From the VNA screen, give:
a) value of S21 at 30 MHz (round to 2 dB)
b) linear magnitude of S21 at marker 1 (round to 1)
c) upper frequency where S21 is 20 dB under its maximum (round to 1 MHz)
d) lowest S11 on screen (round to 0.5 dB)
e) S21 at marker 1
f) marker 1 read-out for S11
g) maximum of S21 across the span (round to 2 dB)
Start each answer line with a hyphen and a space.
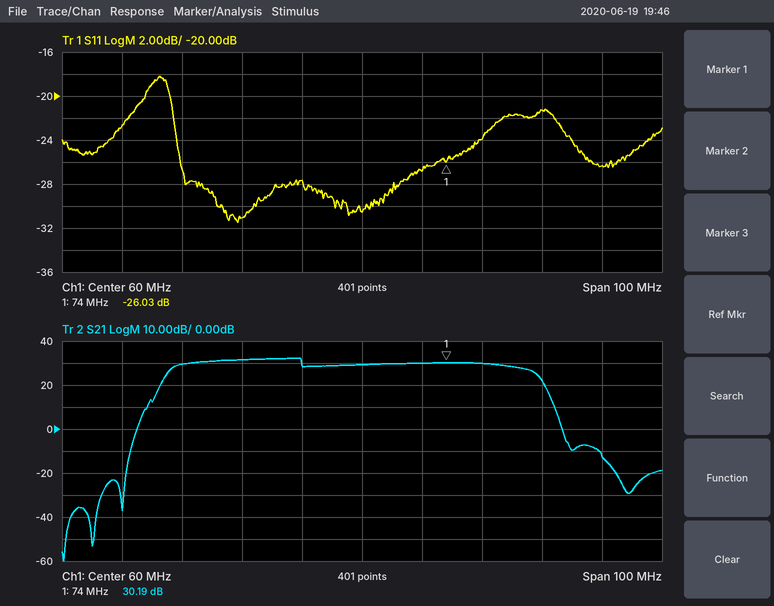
- 30 dB
- 32
- 92 MHz
- -31.5 dB
- 30.19 dB
- -26.03 dB
- 32 dB
